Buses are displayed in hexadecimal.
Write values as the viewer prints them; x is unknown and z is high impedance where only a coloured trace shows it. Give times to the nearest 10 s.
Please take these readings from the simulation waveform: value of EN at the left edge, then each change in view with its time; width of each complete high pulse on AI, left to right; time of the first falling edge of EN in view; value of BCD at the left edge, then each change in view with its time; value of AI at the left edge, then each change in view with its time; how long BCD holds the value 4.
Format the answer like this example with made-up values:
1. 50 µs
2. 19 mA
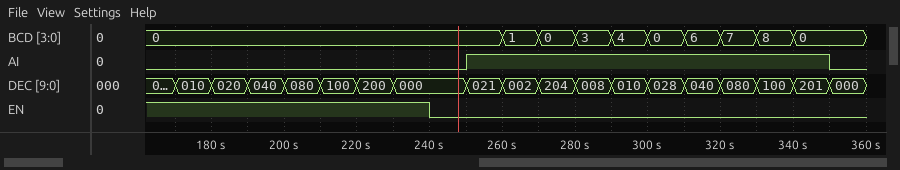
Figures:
1. 1, 0 at 240 s
2. 100 s
3. 240 s
4. 0, 1 at 260 s, 0 at 270 s, 3 at 280 s, 4 at 290 s, 0 at 300 s, 6 at 310 s, 7 at 320 s, 8 at 330 s, 0 at 340 s
5. 0, 1 at 250 s, 0 at 350 s
6. 10 s
